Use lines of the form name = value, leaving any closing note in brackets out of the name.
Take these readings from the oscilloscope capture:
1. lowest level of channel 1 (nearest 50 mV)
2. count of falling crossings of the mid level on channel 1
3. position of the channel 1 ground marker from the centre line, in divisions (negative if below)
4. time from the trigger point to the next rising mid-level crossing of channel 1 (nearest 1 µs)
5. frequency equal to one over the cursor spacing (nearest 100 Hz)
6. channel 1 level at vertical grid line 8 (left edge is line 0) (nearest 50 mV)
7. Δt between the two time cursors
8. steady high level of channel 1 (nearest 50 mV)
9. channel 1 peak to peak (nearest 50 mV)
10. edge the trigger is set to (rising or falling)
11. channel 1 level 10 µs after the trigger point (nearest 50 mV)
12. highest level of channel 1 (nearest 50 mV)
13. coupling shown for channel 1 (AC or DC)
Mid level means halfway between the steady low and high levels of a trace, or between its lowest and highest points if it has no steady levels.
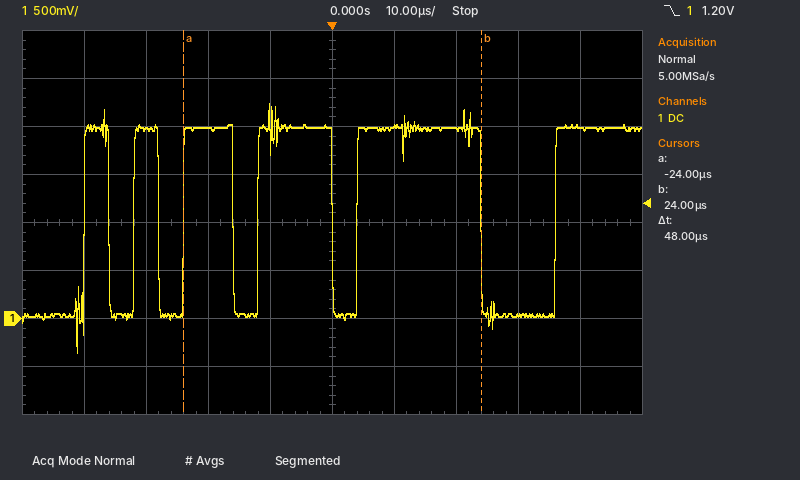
lowest level of channel 1 = -350 mV
count of falling crossings of the mid level on channel 1 = 5
position of the channel 1 ground marker from the centre line, in divisions = -2.0 div
time from the trigger point to the next rising mid-level crossing of channel 1 = 4 µs
frequency equal to one over the cursor spacing = 20.8 kHz
channel 1 level at vertical grid line 8 (left edge is line 0) = 50 mV
Δt between the two time cursors = 48 µs
steady high level of channel 1 = 2.00 V
channel 1 peak to peak = 2.60 V
edge the trigger is set to = falling
channel 1 level 10 µs after the trigger point = 2.00 V
highest level of channel 1 = 2.25 V
coupling shown for channel 1 = DC
